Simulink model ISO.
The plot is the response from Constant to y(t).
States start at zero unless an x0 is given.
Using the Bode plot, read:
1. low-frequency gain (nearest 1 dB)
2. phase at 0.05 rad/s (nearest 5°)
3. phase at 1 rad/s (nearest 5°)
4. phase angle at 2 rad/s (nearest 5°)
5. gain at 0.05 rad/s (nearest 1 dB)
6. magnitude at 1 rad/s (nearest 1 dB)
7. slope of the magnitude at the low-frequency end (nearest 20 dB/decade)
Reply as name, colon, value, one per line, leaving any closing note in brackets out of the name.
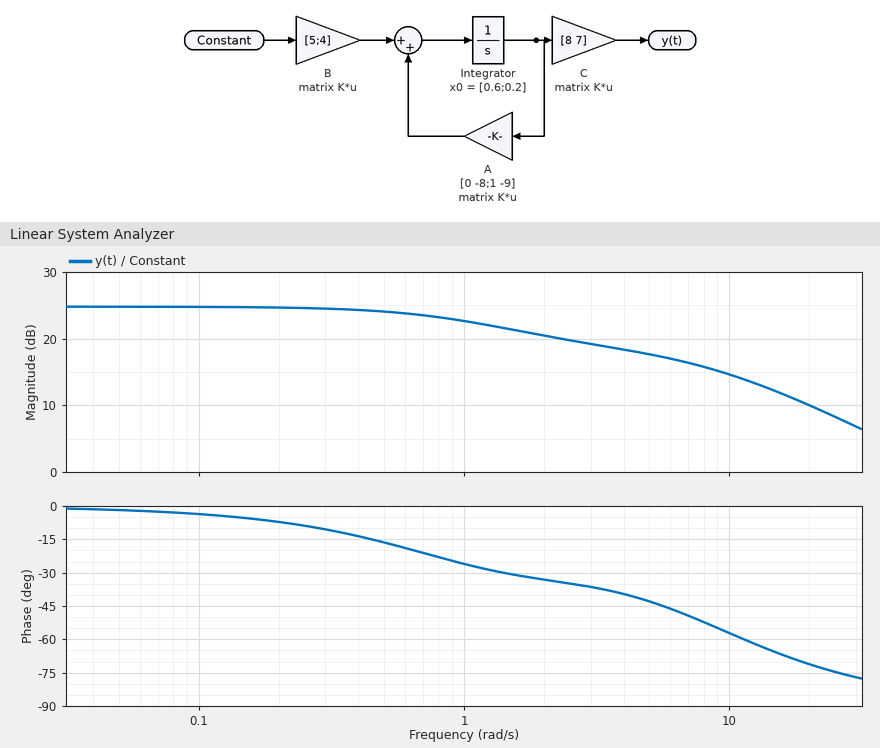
low-frequency gain: 25 dB
phase at 0.05 rad/s: 0°
phase at 1 rad/s: -25°
phase angle at 2 rad/s: -35°
gain at 0.05 rad/s: 25 dB
magnitude at 1 rad/s: 23 dB
slope of the magnitude at the low-frequency end: 0 dB/decade
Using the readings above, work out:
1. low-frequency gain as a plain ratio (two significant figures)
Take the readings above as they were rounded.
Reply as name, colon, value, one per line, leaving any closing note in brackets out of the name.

low-frequency gain as a plain ratio: 18
